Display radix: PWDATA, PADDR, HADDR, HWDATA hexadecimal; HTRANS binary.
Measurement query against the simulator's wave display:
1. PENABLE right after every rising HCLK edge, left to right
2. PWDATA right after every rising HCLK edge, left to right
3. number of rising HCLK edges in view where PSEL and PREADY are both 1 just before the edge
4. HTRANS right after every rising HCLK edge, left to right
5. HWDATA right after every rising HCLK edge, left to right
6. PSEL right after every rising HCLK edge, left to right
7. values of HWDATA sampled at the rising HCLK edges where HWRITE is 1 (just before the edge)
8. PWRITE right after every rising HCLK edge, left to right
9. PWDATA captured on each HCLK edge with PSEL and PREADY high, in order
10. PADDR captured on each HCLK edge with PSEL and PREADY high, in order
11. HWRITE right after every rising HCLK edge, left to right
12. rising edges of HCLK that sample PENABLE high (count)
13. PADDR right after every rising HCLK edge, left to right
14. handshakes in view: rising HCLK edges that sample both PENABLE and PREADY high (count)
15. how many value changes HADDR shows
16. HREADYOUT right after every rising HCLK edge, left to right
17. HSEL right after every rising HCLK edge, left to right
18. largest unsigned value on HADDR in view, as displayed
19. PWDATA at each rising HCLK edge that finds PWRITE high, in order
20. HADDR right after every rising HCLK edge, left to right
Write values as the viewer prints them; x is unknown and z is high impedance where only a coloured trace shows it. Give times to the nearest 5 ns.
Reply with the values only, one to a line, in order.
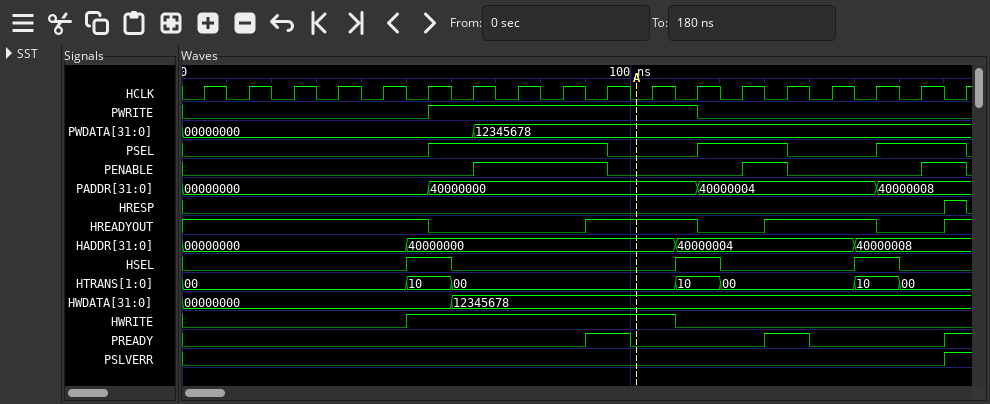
0 0 0 0 0 0 1 1 1 0 0 0 1 0 0 0 1 0
00000000, 00000000, 00000000, 00000000, 00000000, 00000000, 12345678, 12345678, 12345678, 12345678, 12345678, 12345678, 12345678, 12345678, 12345678, 12345678, 12345678, 12345678
3
00, 00, 00, 00, 00, 10, 00, 00, 00, 00, 00, 10, 00, 00, 00, 10, 00, 00
00000000, 00000000, 00000000, 00000000, 00000000, 00000000, 12345678, 12345678, 12345678, 12345678, 12345678, 12345678, 12345678, 12345678, 12345678, 12345678, 12345678, 12345678
0 0 0 0 0 1 1 1 1 0 0 1 1 0 0 1 1 0
00000000, 12345678, 12345678, 12345678, 12345678, 12345678
0 0 0 0 0 1 1 1 1 1 1 0 0 0 0 0 0 0
12345678, 12345678, 12345678
40000000, 40000004, 40000008
0 0 0 0 0 1 1 1 1 1 1 0 0 0 0 0 0 0
5
00000000, 00000000, 00000000, 00000000, 00000000, 40000000, 40000000, 40000000, 40000000, 40000000, 40000000, 40000004, 40000004, 40000004, 40000004, 40000008, 40000008, 40000008
3
3
1 1 1 1 1 0 0 0 0 1 1 0 0 1 1 0 0 1
0 0 0 0 0 1 0 0 0 0 0 1 0 0 0 1 0 0
40000008
00000000, 12345678, 12345678, 12345678, 12345678, 12345678
00000000, 00000000, 00000000, 00000000, 00000000, 40000000, 40000000, 40000000, 40000000, 40000000, 40000000, 40000004, 40000004, 40000004, 40000004, 40000008, 40000008, 40000008
